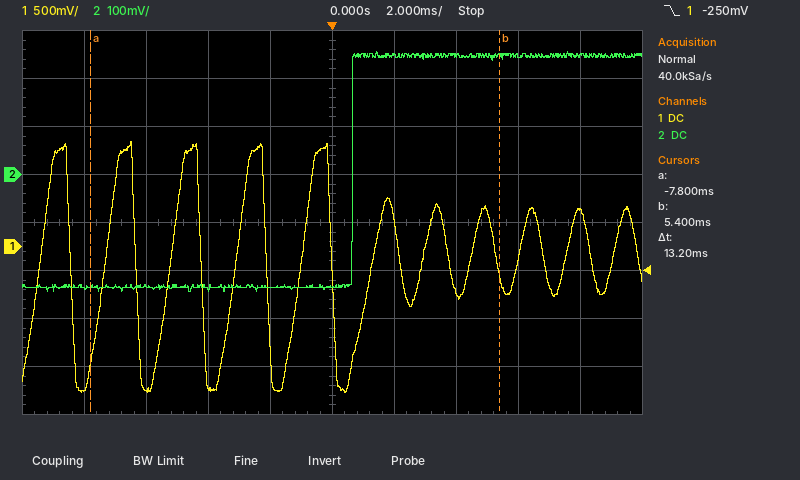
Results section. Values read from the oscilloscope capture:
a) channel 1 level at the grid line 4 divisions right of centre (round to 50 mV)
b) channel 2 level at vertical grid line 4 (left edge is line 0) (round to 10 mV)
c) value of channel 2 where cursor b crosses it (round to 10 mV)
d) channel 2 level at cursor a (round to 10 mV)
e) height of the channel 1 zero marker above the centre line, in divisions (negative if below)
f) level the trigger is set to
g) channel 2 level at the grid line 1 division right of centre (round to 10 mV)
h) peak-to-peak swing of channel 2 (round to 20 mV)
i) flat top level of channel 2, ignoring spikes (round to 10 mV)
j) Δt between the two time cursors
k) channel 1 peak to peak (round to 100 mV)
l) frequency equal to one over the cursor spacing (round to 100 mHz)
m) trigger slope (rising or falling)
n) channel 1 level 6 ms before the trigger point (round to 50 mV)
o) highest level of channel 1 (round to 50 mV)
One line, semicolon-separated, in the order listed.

350 mV; -240 mV; 250 mV; -230 mV; -0.5 div; -250 mV; 250 mV; 500 mV; 250 mV; 13.2 ms; 2.60 V; 75.8 Hz; falling; -1.50 V; 1.10 V
